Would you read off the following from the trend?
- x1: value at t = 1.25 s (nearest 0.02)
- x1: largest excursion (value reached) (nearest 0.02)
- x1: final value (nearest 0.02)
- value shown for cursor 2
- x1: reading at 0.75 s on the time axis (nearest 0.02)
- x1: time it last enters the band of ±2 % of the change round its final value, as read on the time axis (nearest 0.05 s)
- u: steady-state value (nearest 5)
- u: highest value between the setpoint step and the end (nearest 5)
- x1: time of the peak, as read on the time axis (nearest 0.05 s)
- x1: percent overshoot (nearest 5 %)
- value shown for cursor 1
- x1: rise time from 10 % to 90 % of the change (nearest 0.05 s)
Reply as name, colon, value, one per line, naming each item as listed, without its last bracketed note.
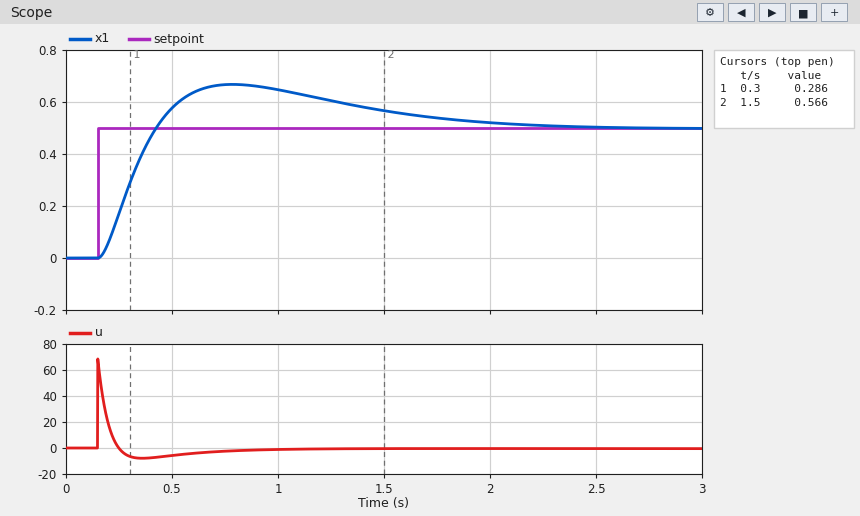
x1: value at t = 1.25 s: 0.60
x1: largest excursion (value reached): 0.66
x1: final value: 0.50
value shown for cursor 2: 0.566
x1: reading at 0.75 s on the time axis: 0.66
x1: time it last enters the band of ±2 % of the change round its final value, as read on the time axis: 2.25 s
u: steady-state value: 0
u: highest value between the setpoint step and the end: 70
x1: time of the peak, as read on the time axis: 0.80 s
x1: percent overshoot: 35 %
value shown for cursor 1: 0.286
x1: rise time from 10 % to 90 % of the change: 0.20 s
